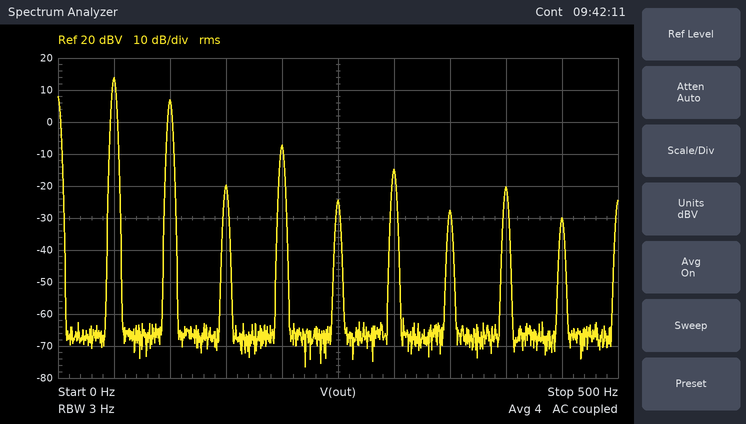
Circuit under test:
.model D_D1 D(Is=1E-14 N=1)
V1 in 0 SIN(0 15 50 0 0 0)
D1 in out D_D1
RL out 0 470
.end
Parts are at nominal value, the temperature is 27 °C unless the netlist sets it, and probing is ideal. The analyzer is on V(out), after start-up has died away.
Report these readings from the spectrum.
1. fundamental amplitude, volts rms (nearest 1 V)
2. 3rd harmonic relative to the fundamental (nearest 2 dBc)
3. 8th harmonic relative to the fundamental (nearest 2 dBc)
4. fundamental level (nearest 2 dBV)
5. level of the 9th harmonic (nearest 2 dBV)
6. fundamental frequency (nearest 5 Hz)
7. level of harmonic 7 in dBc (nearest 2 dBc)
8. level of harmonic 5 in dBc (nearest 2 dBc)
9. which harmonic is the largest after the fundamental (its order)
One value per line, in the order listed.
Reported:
5 V
-34 dBc
-34 dBc
14 dBV
-30 dBV
50 Hz
-42 dBc
-38 dBc
2
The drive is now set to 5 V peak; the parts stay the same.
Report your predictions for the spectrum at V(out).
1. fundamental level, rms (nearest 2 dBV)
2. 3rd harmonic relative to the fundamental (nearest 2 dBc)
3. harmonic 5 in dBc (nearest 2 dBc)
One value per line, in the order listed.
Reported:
4 dBV
-24 dBc
-28 dBc
